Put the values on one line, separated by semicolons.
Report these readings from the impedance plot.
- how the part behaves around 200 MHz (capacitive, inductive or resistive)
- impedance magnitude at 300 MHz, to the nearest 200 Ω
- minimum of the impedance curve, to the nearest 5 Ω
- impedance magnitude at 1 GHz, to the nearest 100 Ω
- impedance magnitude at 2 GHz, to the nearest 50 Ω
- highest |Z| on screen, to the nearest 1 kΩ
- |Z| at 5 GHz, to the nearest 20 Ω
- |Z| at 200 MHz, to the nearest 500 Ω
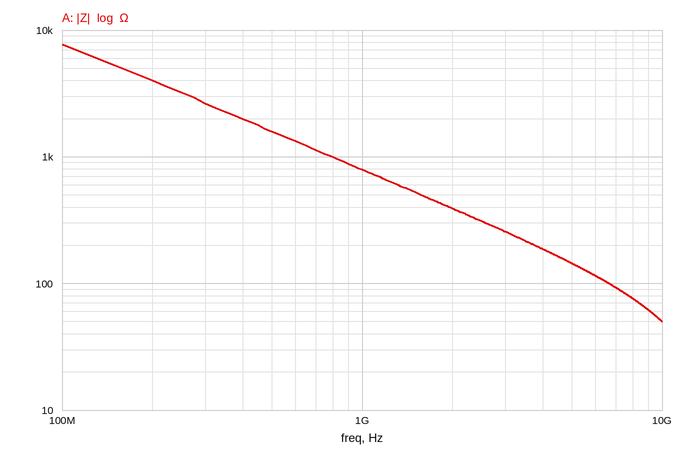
capacitive; 2.6 kΩ; 50 Ω; 800 Ω; 400 Ω; 8 kΩ; 140 Ω; 4.0 kΩ
